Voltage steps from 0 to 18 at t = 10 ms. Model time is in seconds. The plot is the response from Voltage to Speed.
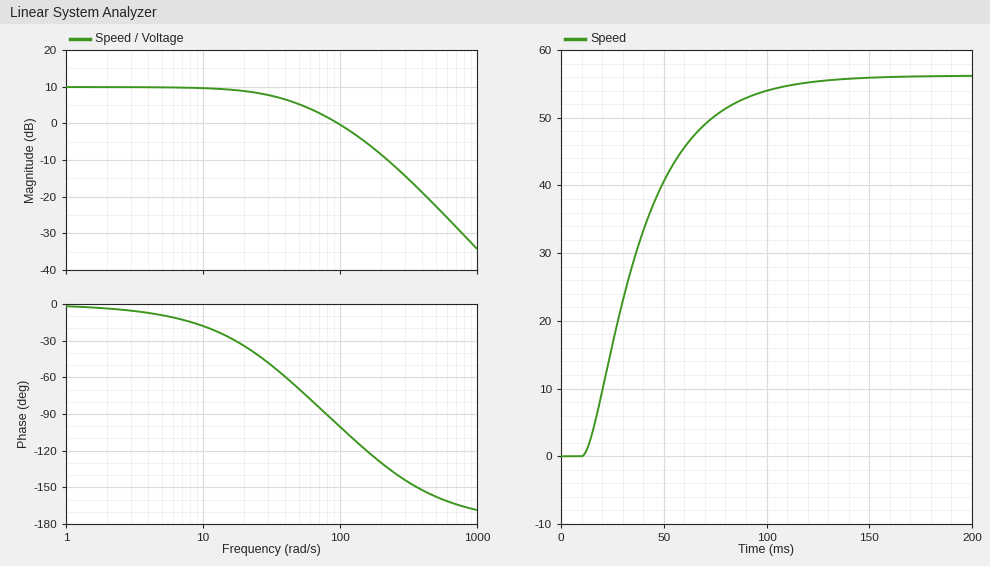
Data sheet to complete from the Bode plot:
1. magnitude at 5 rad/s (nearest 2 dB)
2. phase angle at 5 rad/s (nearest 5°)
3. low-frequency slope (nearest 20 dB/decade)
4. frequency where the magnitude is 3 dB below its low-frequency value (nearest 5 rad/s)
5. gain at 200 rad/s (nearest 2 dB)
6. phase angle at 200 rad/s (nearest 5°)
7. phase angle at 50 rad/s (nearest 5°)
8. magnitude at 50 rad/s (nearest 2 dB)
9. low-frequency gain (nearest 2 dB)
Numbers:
10 dB
-10°
0 dB/decade
35 rad/s
-8 dB
-130°
-70°
6 dB
10 dB
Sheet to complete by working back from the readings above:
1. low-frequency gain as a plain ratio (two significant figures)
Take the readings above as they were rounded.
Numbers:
3.2
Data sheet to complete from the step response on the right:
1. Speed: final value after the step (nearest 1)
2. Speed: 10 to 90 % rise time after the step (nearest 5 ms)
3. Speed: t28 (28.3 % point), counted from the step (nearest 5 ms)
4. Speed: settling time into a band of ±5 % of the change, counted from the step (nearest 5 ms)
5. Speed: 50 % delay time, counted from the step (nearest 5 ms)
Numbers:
56
60 ms
15 ms
85 ms
25 ms
